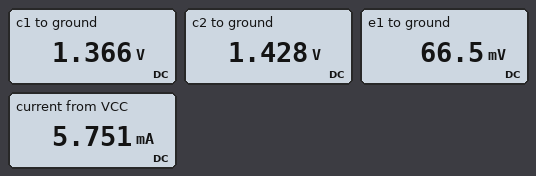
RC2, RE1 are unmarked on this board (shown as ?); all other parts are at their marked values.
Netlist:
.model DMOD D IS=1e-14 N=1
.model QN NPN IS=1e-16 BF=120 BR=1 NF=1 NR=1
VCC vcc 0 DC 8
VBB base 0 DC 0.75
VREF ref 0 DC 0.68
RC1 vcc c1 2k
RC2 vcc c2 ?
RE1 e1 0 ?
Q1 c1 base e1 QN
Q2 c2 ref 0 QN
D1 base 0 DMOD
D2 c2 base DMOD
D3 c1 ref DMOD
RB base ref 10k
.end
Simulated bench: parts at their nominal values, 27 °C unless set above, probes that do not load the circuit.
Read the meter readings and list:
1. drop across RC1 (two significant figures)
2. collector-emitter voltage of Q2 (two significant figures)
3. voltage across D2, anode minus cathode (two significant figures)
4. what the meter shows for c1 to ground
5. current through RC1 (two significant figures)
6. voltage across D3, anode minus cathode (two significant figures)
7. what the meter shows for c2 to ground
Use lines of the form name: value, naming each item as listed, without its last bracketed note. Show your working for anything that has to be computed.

drop across RC1: 8 V - 1.366 V = 6.6 V
collector-emitter voltage of Q2: 1.428 V = 1.4 V
voltage across D2, anode minus cathode: 1.428 V - 750 mV = 680 mV
what the meter shows for c1 to ground: 1.366 V
current through RC1: (8 V - 1.366 V) / 2 kΩ = 3.3 mA
voltage across D3, anode minus cathode: 1.366 V - 680 mV = 690 mV
what the meter shows for c2 to ground: 1.428 V
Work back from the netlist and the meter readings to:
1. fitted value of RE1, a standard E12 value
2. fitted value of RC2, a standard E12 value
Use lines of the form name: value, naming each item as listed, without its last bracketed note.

fitted value of RE1, a standard E12 value: 2.2 kΩ
fitted value of RC2, a standard E12 value: 2.7 kΩ
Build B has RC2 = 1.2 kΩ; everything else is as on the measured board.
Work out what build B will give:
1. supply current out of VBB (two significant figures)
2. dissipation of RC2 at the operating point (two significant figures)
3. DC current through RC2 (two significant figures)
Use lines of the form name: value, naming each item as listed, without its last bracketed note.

supply current out of VBB: 34 mA
dissipation of RC2 at the operating point: 36 mW
DC current through RC2: 5.5 mA
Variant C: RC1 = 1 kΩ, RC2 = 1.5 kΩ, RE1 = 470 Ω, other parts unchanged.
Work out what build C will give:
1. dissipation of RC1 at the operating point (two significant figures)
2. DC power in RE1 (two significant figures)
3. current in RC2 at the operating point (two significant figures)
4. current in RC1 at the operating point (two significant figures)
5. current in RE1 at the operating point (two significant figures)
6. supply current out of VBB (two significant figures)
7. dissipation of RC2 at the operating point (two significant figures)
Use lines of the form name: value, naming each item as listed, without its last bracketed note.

dissipation of RC1 at the operating point: 44 mW
DC power in RE1: 3.4 µW
current in RC2 at the operating point: 4.4 mA
current in RC1 at the operating point: 6.6 mA
current in RE1 at the operating point: 85 µA
supply current out of VBB: 35 mA
dissipation of RC2 at the operating point: 29 mW
